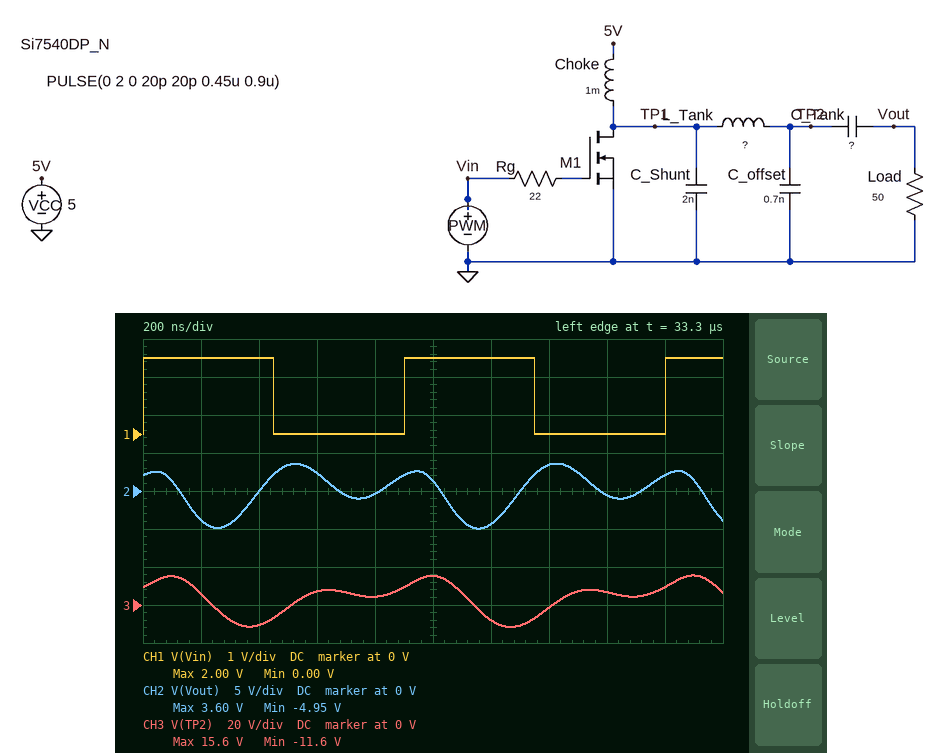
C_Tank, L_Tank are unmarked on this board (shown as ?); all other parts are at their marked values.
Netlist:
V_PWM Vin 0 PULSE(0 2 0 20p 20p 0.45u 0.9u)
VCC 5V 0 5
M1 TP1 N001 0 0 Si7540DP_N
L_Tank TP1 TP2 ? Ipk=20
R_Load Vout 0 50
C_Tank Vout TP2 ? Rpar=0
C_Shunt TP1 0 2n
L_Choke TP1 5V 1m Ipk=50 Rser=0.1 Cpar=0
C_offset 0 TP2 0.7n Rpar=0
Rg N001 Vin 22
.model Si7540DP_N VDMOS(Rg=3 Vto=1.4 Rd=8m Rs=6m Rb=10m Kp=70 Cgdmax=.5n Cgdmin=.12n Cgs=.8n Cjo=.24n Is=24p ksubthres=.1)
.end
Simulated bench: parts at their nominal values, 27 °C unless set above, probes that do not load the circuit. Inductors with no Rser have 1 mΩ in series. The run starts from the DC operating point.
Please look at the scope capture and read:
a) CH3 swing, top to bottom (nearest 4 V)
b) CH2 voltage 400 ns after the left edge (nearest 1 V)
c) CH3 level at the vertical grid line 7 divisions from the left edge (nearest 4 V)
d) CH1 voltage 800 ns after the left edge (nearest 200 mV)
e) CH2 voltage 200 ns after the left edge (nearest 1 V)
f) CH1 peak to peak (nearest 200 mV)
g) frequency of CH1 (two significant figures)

28 V
0 V
0 V
0 V
-4 V
2.0 V
1.1 MHz
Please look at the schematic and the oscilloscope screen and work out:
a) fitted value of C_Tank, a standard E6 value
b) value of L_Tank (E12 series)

680 pF
5.6 µH
